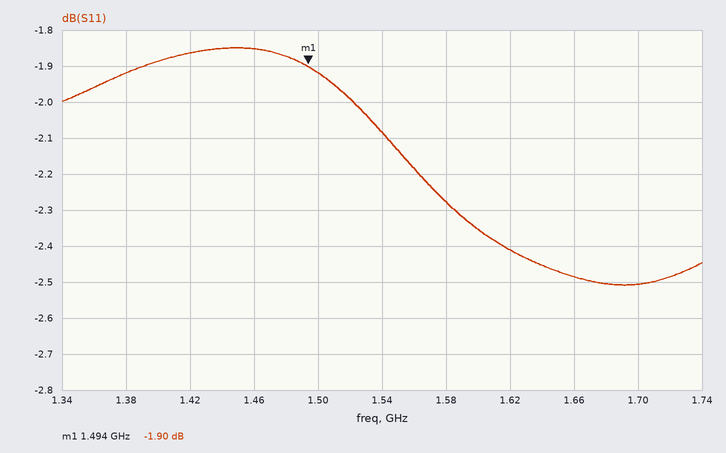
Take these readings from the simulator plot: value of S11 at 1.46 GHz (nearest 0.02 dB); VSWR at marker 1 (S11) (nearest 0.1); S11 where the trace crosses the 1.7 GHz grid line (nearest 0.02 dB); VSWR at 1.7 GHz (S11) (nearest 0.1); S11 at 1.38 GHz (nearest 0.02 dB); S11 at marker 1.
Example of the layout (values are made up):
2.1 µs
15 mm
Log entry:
-1.86 dB
9.2
-2.50 dB
7.0
-1.92 dB
-1.90 dB
